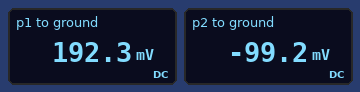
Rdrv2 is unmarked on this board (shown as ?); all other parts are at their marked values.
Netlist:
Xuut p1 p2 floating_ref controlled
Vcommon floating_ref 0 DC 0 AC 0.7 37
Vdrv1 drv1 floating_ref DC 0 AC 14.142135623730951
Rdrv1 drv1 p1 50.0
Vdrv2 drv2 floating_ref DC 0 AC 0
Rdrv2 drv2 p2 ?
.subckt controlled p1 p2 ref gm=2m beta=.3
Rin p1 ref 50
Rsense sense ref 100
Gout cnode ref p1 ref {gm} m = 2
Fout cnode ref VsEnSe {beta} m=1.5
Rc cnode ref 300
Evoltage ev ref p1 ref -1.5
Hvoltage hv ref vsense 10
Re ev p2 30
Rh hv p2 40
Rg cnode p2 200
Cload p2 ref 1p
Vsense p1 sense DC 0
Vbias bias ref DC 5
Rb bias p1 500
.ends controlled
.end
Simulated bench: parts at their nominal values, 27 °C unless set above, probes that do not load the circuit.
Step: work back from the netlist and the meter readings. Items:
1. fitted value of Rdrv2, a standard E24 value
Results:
24 Ω
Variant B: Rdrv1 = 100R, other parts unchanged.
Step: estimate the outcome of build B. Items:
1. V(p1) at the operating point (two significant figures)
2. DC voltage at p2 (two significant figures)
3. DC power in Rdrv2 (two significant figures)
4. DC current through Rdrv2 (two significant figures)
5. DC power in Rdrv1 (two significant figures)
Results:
240 mV
-120 mV
630 µW
5.1 mA
570 µW
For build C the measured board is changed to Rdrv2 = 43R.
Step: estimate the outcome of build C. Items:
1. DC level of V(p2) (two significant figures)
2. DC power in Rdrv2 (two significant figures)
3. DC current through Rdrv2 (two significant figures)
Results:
-120 mV
340 µW
2.8 mA
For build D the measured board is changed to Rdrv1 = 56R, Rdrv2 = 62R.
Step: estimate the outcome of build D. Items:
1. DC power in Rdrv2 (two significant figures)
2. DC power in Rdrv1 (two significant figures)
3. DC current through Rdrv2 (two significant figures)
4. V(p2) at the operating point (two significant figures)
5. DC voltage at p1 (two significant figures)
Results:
310 µW
720 µW
2.2 mA
-140 mV
200 mV
